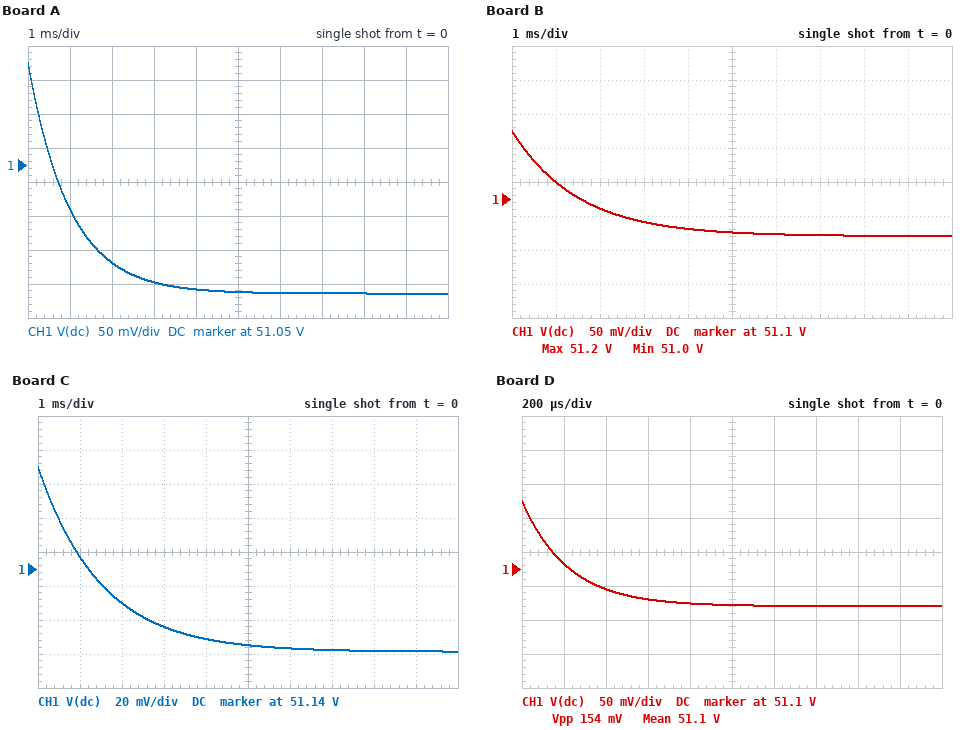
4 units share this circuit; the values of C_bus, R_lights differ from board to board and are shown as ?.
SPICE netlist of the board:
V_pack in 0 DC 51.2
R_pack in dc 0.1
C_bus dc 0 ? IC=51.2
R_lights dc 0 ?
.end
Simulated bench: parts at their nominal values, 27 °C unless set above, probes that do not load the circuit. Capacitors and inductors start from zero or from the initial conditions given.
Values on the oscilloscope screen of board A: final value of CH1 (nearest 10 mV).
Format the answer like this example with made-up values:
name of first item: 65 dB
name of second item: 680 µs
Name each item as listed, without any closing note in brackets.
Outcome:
final value of CH1: 50.86 V
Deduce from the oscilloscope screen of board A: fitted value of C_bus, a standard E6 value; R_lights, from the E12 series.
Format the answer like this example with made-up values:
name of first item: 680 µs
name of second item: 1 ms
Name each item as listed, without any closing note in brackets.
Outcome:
fitted value of C_bus, a standard E6 value: 10 mF
R_lights, from the E12 series: 15 Ω
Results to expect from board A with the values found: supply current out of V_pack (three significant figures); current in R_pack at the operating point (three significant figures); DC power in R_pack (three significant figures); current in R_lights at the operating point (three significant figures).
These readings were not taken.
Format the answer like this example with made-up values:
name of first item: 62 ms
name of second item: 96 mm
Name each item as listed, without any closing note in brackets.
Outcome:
supply current out of V_pack: 3.39 A
current in R_pack at the operating point: 3.39 A
DC power in R_pack: 1.15 W
current in R_lights at the operating point: 3.39 A
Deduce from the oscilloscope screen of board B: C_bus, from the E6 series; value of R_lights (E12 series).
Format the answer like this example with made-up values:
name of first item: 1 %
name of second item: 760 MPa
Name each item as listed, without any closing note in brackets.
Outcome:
C_bus, from the E6 series: 15 mF
value of R_lights: 33 Ω
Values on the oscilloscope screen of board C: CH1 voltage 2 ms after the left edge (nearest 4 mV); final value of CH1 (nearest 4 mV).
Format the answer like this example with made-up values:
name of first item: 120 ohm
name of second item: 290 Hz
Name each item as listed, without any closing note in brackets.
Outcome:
CH1 voltage 2 ms after the left edge: 51.120 V
final value of CH1: 51.092 V
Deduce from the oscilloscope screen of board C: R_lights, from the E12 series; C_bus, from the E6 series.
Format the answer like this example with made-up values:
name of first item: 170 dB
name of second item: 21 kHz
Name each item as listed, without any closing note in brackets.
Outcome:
R_lights, from the E12 series: 47 Ω
C_bus, from the E6 series: 15 mF
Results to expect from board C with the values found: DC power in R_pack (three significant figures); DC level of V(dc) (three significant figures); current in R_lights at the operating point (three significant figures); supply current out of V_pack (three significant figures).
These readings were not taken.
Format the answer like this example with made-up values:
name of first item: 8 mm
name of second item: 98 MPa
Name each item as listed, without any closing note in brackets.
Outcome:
DC power in R_pack: 118 mW
DC level of V(dc): 51.1 V
current in R_lights at the operating point: 1.09 A
supply current out of V_pack: 1.09 A
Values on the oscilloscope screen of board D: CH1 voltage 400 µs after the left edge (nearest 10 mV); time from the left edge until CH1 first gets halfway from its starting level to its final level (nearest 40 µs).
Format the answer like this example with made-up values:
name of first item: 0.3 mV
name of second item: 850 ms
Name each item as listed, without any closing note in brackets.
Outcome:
CH1 voltage 400 µs after the left edge: 51.07 V
time from the left edge until CH1 first gets halfway from its starting level to its final level: 160 µs
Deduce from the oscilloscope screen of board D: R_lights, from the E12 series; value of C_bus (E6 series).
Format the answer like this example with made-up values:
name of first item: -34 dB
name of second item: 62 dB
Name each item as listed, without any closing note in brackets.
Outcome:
R_lights, from the E12 series: 33 Ω
value of C_bus: 2.2 mF
